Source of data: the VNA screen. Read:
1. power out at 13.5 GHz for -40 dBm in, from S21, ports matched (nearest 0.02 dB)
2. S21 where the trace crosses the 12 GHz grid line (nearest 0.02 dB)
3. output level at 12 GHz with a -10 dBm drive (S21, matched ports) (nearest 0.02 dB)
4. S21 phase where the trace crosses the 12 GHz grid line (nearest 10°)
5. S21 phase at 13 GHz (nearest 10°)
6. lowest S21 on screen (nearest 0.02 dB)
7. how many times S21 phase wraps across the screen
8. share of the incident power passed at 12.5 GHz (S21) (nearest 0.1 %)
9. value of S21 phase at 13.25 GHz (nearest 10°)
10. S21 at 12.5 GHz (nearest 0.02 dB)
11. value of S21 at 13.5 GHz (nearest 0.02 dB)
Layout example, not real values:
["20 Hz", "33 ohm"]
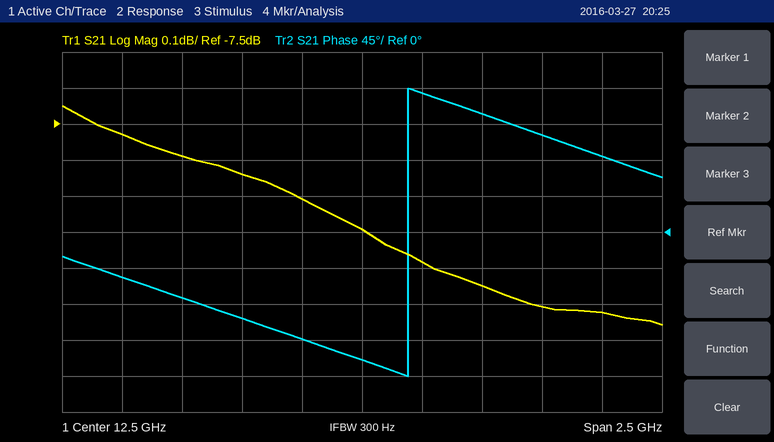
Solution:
["-48.02 dBm", "-7.64 dB", "-17.64 dBm", "-110°", "150°", "-8.06 dB", "1", "16.6 %", "120°", "-7.80 dB", "-8.02 dB"]
